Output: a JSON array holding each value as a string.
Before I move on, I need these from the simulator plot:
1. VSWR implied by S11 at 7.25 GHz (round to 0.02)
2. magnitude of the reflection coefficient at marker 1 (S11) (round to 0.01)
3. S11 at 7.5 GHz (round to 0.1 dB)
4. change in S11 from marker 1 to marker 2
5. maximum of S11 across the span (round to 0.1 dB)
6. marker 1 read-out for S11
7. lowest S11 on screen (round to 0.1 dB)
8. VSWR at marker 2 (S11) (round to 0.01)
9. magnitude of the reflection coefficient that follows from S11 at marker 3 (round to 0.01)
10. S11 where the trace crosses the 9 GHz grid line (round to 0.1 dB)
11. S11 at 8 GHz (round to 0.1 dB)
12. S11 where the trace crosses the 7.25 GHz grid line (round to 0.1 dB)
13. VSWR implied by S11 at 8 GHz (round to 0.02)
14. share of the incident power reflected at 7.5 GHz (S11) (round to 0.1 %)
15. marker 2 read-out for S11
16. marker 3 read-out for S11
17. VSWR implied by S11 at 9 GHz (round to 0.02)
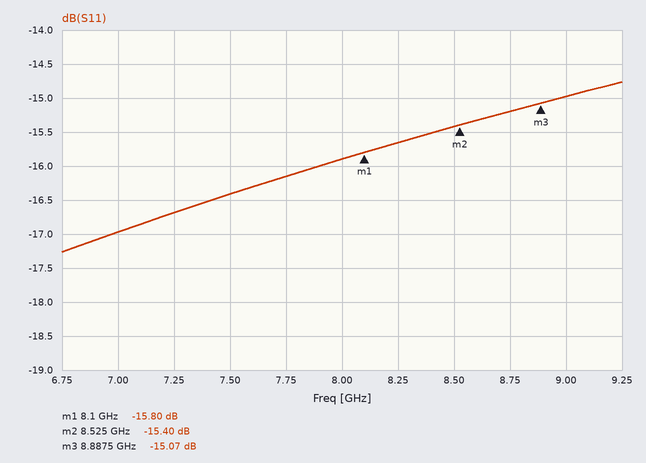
["1.34", "0.16", "-16.4 dB", "0.40 dB", "-14.8 dB", "-15.80 dB", "-17.3 dB", "1.41", "0.18", "-15.0 dB", "-15.9 dB", "-16.7 dB", "1.38", "2.3 %", "-15.40 dB", "-15.07 dB", "1.44"]
